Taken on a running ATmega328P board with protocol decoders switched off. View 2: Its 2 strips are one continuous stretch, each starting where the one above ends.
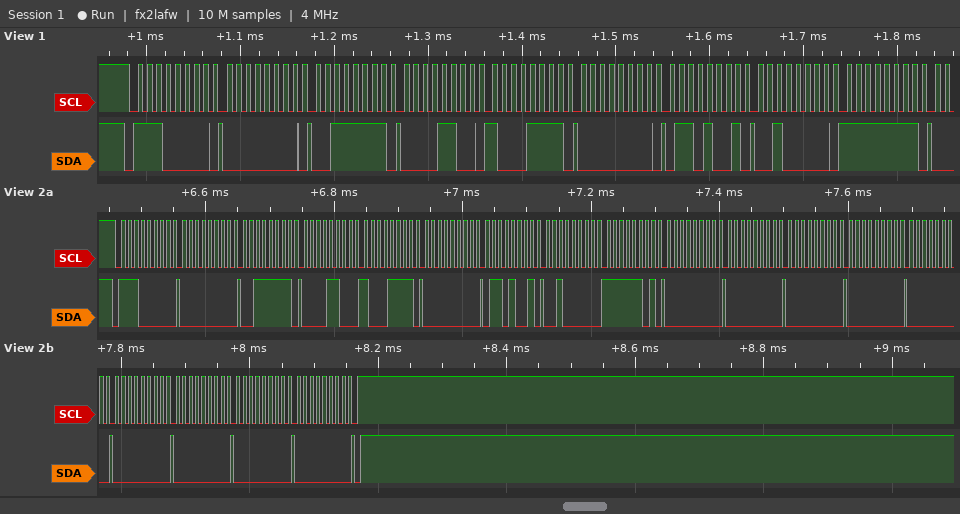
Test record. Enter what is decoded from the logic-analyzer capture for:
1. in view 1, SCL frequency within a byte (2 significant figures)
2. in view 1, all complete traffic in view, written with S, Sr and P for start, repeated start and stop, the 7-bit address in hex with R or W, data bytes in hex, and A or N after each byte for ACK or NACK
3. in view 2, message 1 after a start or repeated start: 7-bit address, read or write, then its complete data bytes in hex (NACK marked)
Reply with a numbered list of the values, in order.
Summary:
1. 100 kHz
2. S 70W A 00 A 3F A 0C A 8F A 00 A 69 A 20 A FF A
3. 0x70 write: 00 3F 0C 8F 00 69 20 FD 00 00 00 00 00 00 00 00 00
